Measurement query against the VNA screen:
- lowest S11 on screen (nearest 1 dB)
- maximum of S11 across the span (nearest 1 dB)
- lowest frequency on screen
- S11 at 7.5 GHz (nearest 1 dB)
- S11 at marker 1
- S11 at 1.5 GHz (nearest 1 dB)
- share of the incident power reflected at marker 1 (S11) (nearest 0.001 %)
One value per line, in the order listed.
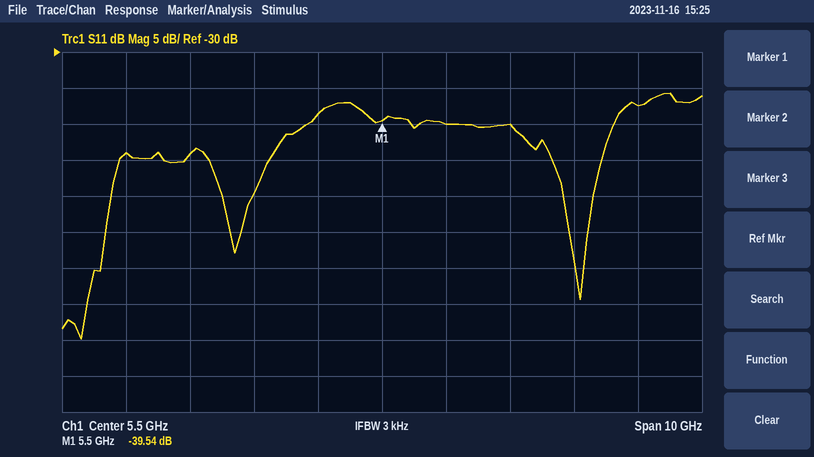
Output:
-70 dB
-36 dB
500 MHz
-40 dB
-39.54 dB
-44 dB
0.011 %
